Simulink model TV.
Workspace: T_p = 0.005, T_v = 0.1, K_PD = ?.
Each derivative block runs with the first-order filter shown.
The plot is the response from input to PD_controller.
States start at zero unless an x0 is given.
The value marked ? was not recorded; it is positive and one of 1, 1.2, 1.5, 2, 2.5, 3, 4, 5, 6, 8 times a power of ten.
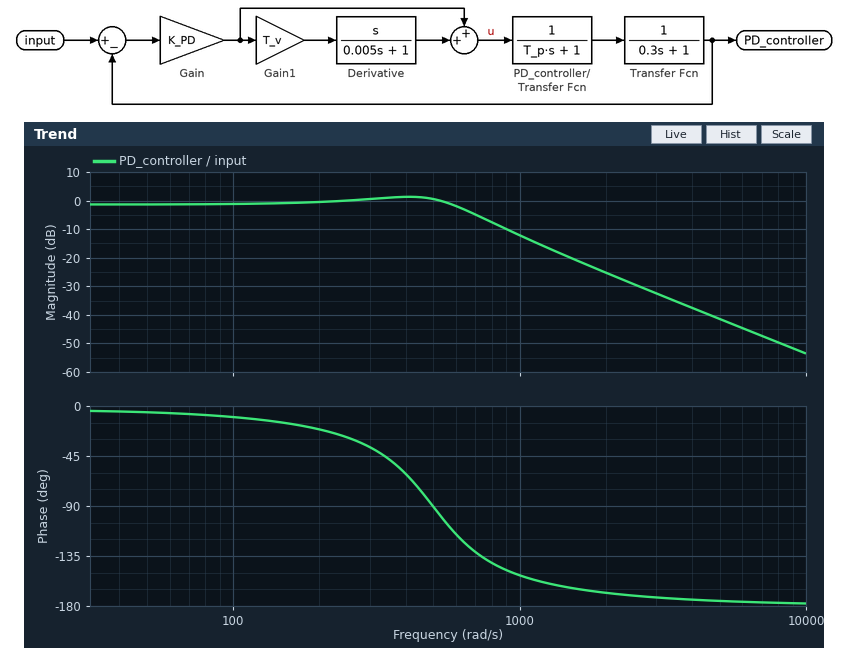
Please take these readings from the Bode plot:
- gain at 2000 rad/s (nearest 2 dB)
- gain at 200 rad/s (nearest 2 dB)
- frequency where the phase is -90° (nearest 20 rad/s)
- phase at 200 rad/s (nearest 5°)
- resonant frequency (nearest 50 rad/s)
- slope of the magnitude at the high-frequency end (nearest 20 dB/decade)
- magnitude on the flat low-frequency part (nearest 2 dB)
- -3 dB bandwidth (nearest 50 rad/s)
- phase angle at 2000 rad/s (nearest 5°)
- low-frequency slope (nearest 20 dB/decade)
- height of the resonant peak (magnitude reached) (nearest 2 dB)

-26 dB
0 dB
500 rad/s
-20°
400 rad/s
-40 dB/decade
-2 dB
700 rad/s
-170°
0 dB/decade
2 dB
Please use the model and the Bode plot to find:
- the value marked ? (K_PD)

15
